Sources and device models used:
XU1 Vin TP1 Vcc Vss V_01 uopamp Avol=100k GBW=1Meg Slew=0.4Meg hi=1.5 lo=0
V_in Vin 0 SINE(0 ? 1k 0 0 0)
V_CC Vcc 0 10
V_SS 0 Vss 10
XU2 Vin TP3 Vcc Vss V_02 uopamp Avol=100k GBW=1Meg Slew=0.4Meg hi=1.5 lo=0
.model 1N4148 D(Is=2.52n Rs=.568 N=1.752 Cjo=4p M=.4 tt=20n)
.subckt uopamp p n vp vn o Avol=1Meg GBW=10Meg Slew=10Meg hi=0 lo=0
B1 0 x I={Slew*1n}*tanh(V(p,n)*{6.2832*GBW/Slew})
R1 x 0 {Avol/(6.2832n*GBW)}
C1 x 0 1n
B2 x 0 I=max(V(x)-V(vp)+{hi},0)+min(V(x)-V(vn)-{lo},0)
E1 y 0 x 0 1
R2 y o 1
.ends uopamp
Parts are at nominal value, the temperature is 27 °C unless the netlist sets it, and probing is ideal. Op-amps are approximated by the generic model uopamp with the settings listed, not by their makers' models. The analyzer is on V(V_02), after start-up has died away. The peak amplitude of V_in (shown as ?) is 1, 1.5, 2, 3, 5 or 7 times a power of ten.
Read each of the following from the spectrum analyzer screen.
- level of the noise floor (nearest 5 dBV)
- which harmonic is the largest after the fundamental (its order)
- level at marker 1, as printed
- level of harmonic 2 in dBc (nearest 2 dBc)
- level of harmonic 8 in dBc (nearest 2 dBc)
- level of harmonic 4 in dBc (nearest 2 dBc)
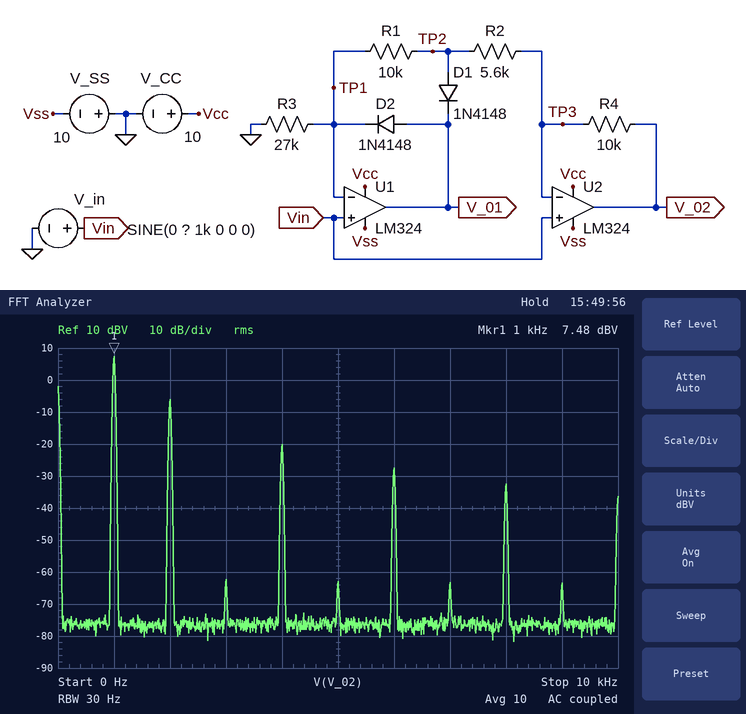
-75 dBV
2
7.48 dBV
-14 dBc
-40 dBc
-28 dBc
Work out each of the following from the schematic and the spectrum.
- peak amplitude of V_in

5 V
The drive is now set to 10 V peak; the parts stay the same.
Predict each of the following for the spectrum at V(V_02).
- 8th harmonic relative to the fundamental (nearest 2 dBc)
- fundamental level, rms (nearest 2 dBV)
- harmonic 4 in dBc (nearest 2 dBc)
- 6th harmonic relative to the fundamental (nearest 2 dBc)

-34 dBc
16 dBV
-18 dBc
-32 dBc
